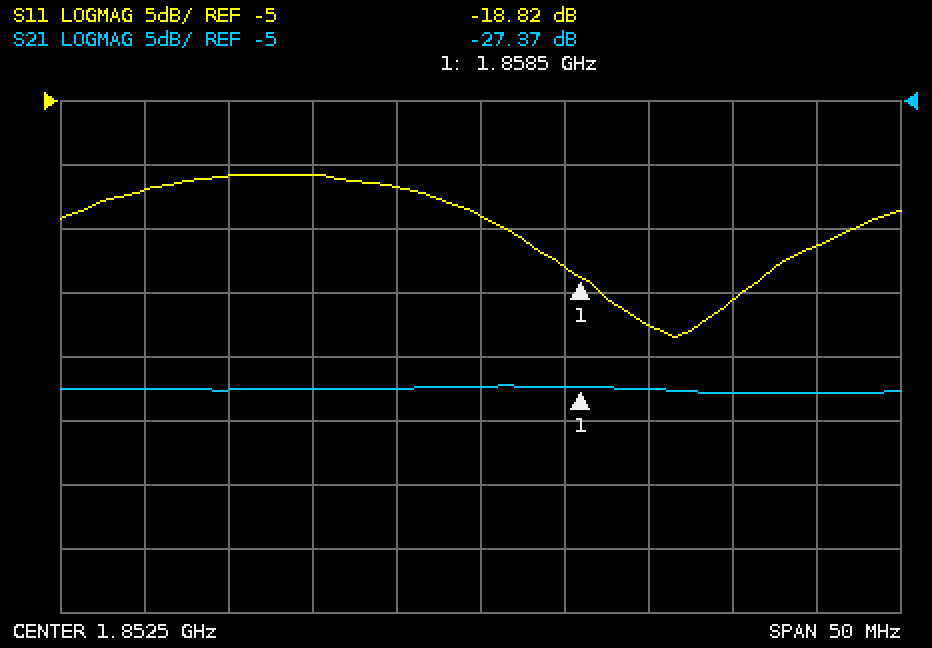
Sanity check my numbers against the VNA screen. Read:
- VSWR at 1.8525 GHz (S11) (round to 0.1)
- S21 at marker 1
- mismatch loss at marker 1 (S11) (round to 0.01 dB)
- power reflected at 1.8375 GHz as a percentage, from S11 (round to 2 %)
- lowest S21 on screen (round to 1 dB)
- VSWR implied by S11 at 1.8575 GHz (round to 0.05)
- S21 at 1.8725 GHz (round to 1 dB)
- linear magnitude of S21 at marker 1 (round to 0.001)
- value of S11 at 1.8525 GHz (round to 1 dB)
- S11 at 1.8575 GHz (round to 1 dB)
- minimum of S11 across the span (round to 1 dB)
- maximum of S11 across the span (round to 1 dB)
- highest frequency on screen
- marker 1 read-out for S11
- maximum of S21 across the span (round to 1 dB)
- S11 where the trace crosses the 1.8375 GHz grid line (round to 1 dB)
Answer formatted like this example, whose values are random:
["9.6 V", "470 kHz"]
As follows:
["1.5", "-27.37 dB", "0.06 dB", "8 %", "-28 dB", "1.30", "-28 dB", "0.043", "-14 dB", "-18 dB", "-23 dB", "-11 dB", "1.8775 GHz", "-18.82 dB", "-27 dB", "-11 dB"]
